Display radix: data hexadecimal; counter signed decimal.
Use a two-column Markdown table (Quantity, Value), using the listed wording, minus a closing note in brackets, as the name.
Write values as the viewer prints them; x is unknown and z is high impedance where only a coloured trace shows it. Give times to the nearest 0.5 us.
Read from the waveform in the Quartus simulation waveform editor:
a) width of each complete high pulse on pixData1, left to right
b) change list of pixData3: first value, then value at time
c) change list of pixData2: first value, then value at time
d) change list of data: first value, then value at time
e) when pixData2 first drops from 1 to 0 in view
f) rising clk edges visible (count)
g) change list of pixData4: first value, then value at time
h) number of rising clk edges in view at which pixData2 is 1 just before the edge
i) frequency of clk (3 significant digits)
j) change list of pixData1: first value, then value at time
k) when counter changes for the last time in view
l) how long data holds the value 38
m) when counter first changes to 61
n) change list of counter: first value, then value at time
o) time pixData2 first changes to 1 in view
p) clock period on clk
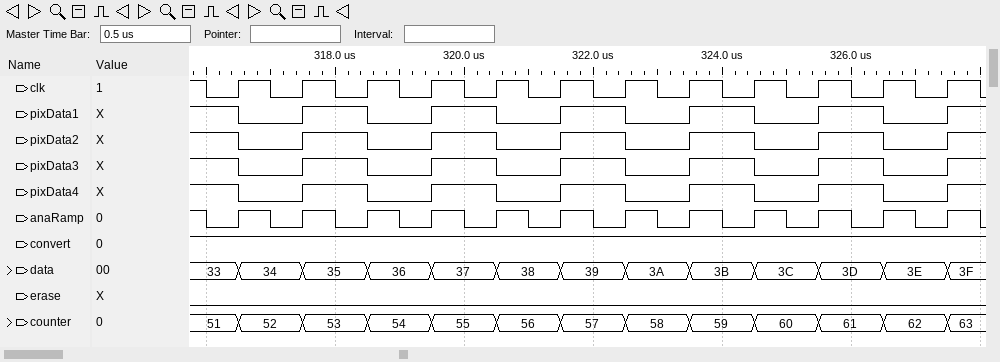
| Quantity | Value |
|---|---|
| width of each complete high pulse on pixData1, left to right | 1 us, 1 us, 1 us, 1 us, 1 us |
| change list of pixData3: first value, then value at time | 1, 0 at 316.5 us, 1 at 317.5 us, 0 at 318.5 us, 1 at 319.5 us, 0 at 320.5 us, 1 at 321.5 us, 0 at 322.5 us, 1 at 323.5 us, 0 at 324.5 us, 1 at 325.5 us, 0 at 326.5 us, 1 at 327.5 us |
| change list of pixData2: first value, then value at time | 1, 0 at 316.5 us, 1 at 317.5 us, 0 at 318.5 us, 1 at 319.5 us, 0 at 320.5 us, 1 at 321.5 us, 0 at 322.5 us, 1 at 323.5 us, 0 at 324.5 us, 1 at 325.5 us, 0 at 326.5 us, 1 at 327.5 us |
| change list of data: first value, then value at time | 33, 34 at 316.5 us, 35 at 317.5 us, 36 at 318.5 us, 37 at 319.5 us, 38 at 320.5 us, 39 at 321.5 us, 3A at 322.5 us, 3B at 323.5 us, 3C at 324.5 us, 3D at 325.5 us, 3E at 326.5 us, 3F at 327.5 us |
| when pixData2 first drops from 1 to 0 in view | 316.5 us |
| rising clk edges visible | 12 |
| change list of pixData4: first value, then value at time | 1, 0 at 316.5 us, 1 at 317.5 us, 0 at 318.5 us, 1 at 319.5 us, 0 at 320.5 us, 1 at 321.5 us, 0 at 322.5 us, 1 at 323.5 us, 0 at 324.5 us, 1 at 325.5 us, 0 at 326.5 us, 1 at 327.5 us |
| number of rising clk edges in view at which pixData2 is 1 just before the edge | 6 |
| frequency of clk | 1.00 MHz |
| change list of pixData1: first value, then value at time | 1, 0 at 316.5 us, 1 at 317.5 us, 0 at 318.5 us, 1 at 319.5 us, 0 at 320.5 us, 1 at 321.5 us, 0 at 322.5 us, 1 at 323.5 us, 0 at 324.5 us, 1 at 325.5 us, 0 at 326.5 us, 1 at 327.5 us |
| when counter changes for the last time in view | 327.5 us |
| how long data holds the value 38 | 1 us |
| when counter first changes to 61 | 325.5 us |
| change list of counter: first value, then value at time | 51, 52 at 316.5 us, 53 at 317.5 us, 54 at 318.5 us, 55 at 319.5 us, 56 at 320.5 us, 57 at 321.5 us, 58 at 322.5 us, 59 at 323.5 us, 60 at 324.5 us, 61 at 325.5 us, 62 at 326.5 us, 63 at 327.5 us |
| time pixData2 first changes to 1 in view | 317.5 us |
| clock period on clk | 1 us |
